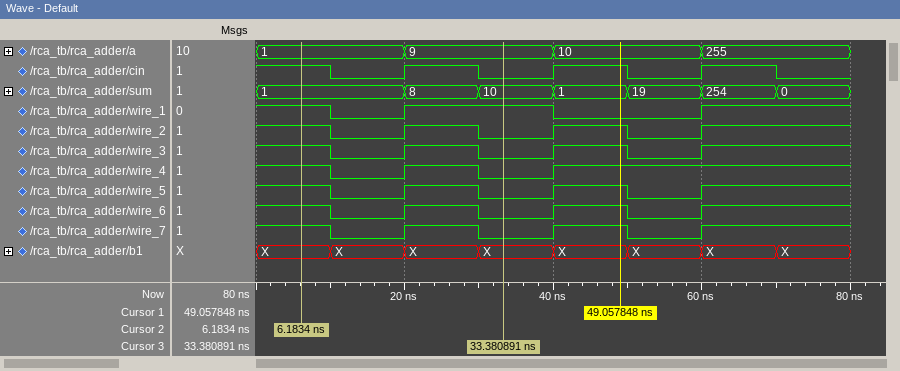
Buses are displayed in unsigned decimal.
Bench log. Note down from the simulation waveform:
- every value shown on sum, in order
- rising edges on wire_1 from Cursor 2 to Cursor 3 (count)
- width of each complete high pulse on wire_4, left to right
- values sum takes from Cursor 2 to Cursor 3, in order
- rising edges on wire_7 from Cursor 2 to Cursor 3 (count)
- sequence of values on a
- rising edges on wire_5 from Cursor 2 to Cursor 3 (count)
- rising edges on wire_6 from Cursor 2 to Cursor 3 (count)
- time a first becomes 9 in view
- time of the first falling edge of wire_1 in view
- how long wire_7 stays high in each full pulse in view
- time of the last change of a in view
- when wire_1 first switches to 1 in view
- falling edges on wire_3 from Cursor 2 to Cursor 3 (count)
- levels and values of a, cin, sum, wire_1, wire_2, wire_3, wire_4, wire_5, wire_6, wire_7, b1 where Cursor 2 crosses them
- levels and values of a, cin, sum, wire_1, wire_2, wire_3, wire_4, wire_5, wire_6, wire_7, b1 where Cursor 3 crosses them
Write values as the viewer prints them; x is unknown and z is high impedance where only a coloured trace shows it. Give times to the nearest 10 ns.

1, 8, 10, 1, 19, 254, 0
1
10 ns
1, 8, 10
1
1, 9, 10, 255
1
1
20 ns
10 ns
10 ns, 10 ns
60 ns
20 ns
2
a=1, cin=1, sum=1, wire_1=1, wire_2=1, wire_3=1, wire_4=1, wire_5=1, wire_6=1, wire_7=1, b1=X
a=9, cin=0, sum=10, wire_1=1, wire_2=0, wire_3=0, wire_4=0, wire_5=0, wire_6=0, wire_7=0, b1=X
